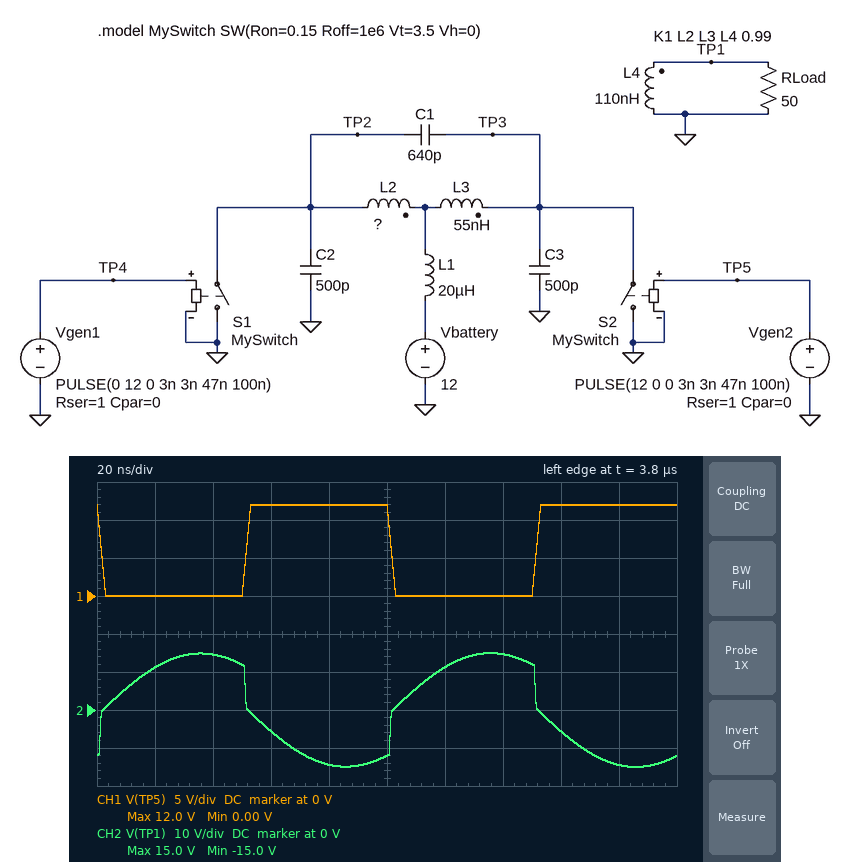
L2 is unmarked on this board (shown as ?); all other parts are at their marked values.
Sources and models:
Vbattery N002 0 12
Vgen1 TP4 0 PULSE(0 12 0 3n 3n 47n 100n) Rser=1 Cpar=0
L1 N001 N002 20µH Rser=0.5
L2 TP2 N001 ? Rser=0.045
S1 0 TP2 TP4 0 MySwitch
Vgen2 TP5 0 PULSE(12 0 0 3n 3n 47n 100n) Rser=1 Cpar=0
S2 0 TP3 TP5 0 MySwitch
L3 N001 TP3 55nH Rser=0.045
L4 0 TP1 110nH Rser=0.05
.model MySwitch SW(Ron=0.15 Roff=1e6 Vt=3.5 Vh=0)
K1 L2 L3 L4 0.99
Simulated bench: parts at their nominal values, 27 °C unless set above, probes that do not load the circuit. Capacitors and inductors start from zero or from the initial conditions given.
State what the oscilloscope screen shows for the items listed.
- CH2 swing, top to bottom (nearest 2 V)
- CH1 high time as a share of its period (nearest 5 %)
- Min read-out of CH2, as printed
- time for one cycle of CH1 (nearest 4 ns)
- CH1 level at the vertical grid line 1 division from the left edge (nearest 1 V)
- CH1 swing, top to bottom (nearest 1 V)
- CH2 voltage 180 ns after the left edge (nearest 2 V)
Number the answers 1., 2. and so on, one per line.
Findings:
1. 30 V
2. 50 %
3. -15.0 V
4. 100 ns
5. 0 V
6. 12 V
7. -14 V
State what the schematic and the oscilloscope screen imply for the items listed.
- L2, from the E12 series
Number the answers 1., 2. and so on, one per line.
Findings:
1. 180 nH
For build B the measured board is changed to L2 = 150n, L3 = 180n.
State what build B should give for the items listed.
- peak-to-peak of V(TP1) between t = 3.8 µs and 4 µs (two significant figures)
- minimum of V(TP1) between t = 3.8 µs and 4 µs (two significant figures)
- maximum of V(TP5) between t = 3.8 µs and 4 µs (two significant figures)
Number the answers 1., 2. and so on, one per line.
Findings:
1. 23 V
2. -12 V
3. 12 V
